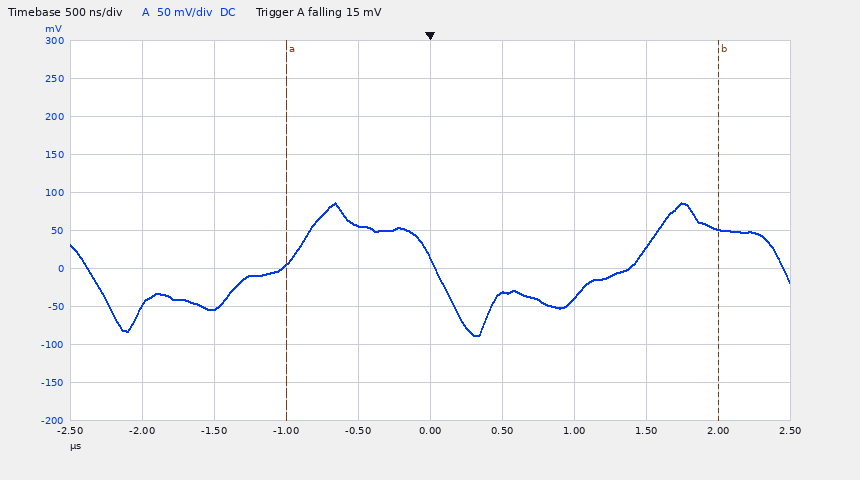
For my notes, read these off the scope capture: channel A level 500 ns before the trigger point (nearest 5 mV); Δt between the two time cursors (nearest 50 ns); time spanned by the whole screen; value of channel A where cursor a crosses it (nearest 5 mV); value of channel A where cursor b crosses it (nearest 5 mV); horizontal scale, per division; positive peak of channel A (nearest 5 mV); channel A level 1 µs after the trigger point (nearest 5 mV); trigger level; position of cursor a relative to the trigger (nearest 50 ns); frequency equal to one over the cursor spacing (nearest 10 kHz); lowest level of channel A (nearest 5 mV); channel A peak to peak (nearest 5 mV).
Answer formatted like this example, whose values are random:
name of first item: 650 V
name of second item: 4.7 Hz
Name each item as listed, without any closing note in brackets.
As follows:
channel A level 500 ns before the trigger point: 55 mV
Δt between the two time cursors: 3.00 µs
time spanned by the whole screen: 5 µs
value of channel A where cursor a crosses it: 5 mV
value of channel A where cursor b crosses it: 50 mV
horizontal scale, per division: 500 ns
positive peak of channel A: 85 mV
channel A level 1 µs after the trigger point: -40 mV
trigger level: 15 mV
position of cursor a relative to the trigger: -1.00 µs
frequency equal to one over the cursor spacing: 330 kHz
lowest level of channel A: -90 mV
channel A peak to peak: 175 mV
